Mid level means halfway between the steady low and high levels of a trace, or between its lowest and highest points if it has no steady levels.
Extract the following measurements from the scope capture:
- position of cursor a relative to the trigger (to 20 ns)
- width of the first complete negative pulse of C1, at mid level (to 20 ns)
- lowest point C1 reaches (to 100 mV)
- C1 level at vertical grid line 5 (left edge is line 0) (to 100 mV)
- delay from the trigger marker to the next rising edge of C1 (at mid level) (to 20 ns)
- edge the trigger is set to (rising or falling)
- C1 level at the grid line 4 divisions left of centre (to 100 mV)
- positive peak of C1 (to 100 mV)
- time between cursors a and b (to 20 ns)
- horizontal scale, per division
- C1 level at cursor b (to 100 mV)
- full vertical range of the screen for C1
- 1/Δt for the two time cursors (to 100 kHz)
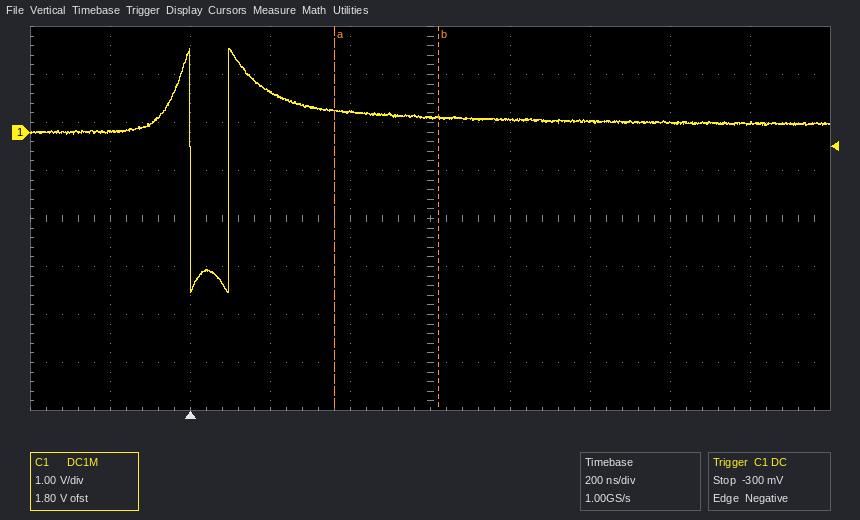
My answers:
+360 ns
100 ns
-3.3 V
300 mV
100 ns
falling
0.0 V
1.7 V
260 ns
200 ns
300 mV
8 V
3.8 MHz
